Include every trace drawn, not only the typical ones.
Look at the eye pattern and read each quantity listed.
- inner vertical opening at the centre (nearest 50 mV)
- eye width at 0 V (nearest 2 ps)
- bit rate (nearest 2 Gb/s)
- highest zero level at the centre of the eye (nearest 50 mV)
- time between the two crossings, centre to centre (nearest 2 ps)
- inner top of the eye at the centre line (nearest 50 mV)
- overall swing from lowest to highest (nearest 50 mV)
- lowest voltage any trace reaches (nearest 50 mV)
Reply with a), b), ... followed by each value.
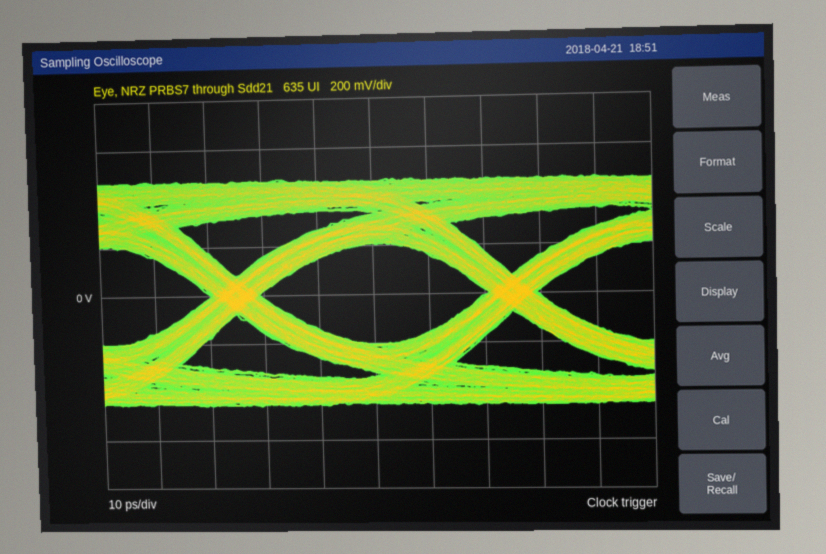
a) 400 mV
b) 42 ps
c) 20 Gb/s
d) -200 mV
e) 50 ps
f) 200 mV
g) 950 mV
h) -450 mV
